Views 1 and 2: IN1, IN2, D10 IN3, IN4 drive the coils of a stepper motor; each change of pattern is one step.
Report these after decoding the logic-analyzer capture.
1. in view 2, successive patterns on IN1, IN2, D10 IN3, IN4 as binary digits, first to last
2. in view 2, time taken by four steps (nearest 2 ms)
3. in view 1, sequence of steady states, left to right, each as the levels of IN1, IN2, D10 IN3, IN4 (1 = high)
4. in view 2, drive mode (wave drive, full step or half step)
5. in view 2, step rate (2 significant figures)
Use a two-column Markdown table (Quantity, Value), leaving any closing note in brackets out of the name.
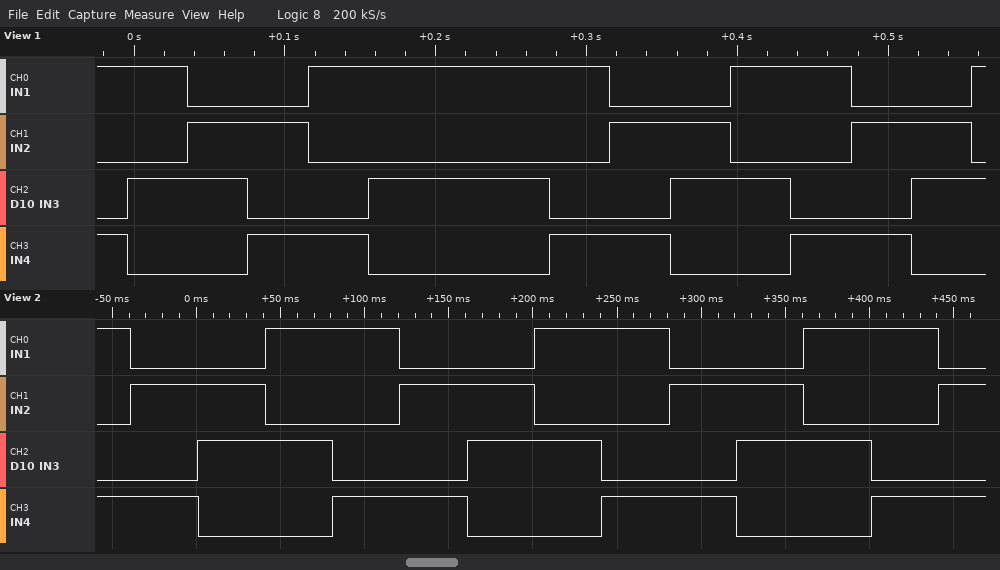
| Quantity | Value |
|---|---|
| in view 2, successive patterns on IN1, IN2, D10 IN3, IN4 as binary digits, first to last | 1001 0101 0110 1010 1001 0101 0110 1010 1001 0101 0110 1010 1001 0101 |
| in view 2, time taken by four steps | 160 ms |
| in view 1, sequence of steady states, left to right, each as the levels of IN1, IN2, D10 IN3, IN4 | 1001 1010 0110 0101 1001 1010 1001 0101 0110 1010 1001 0101 0110 1010 |
| in view 2, drive mode | full step |
| in view 2, step rate | 25 steps/s |
